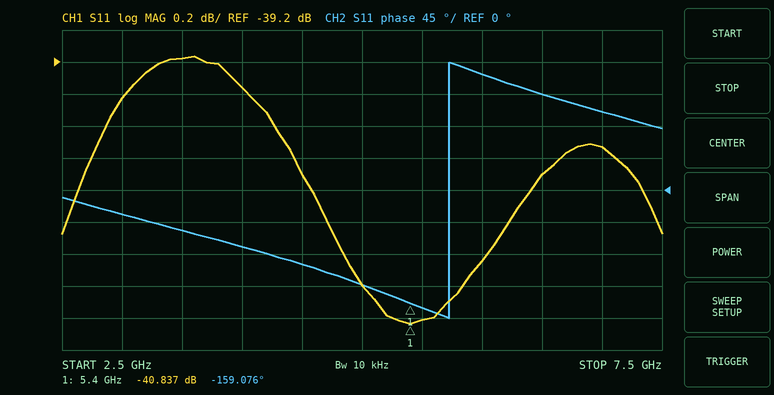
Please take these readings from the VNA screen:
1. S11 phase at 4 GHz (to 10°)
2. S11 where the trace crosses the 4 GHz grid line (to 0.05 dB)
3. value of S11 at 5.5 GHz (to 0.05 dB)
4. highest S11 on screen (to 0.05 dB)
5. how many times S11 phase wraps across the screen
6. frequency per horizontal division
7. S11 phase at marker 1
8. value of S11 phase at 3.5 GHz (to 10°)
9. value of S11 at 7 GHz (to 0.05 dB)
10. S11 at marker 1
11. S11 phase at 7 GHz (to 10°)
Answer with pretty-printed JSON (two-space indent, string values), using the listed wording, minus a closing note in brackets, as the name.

{
  "S11 phase at 4 GHz": "-80°",
  "S11 where the trace crosses the 4 GHz grid line": "-39.35 dB",
  "value of S11 at 5.5 GHz": "-40.80 dB",
  "highest S11 on screen": "-39.15 dB",
  "how many times S11 phase wraps across the screen": "1",
  "frequency per horizontal division": "500 MHz",
  "S11 phase at marker 1": "-159.076°",
  "value of S11 phase at 3.5 GHz": "-60°",
  "value of S11 at 7 GHz": "-39.75 dB",
  "S11 at marker 1": "-40.837 dB",
  "S11 phase at 7 GHz": "110°"
}
